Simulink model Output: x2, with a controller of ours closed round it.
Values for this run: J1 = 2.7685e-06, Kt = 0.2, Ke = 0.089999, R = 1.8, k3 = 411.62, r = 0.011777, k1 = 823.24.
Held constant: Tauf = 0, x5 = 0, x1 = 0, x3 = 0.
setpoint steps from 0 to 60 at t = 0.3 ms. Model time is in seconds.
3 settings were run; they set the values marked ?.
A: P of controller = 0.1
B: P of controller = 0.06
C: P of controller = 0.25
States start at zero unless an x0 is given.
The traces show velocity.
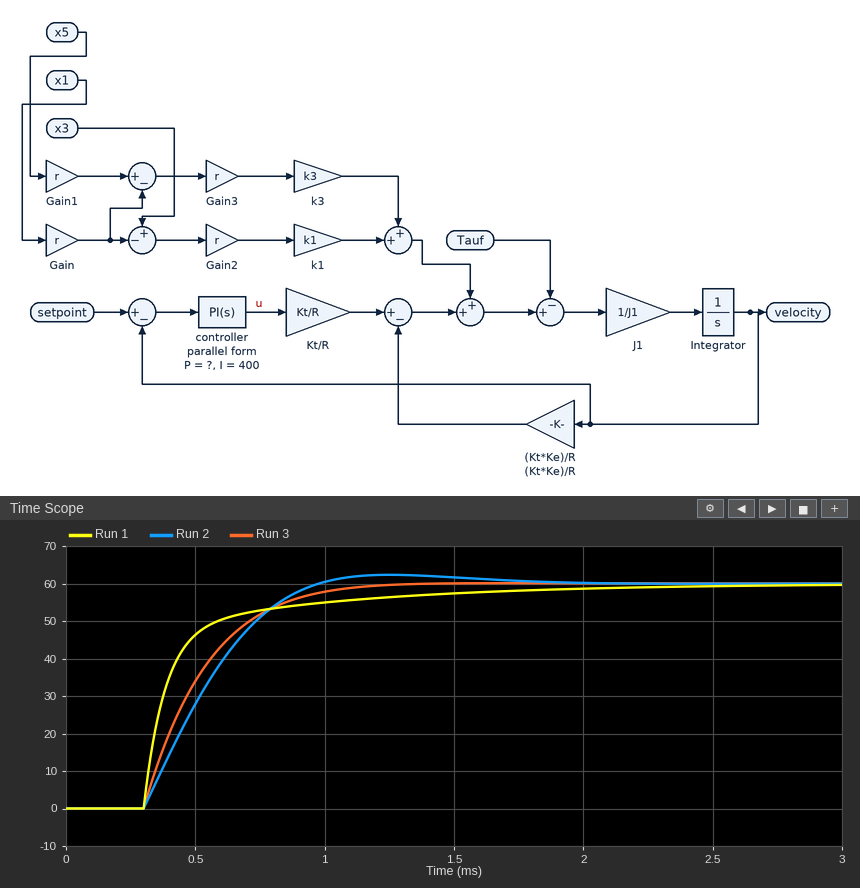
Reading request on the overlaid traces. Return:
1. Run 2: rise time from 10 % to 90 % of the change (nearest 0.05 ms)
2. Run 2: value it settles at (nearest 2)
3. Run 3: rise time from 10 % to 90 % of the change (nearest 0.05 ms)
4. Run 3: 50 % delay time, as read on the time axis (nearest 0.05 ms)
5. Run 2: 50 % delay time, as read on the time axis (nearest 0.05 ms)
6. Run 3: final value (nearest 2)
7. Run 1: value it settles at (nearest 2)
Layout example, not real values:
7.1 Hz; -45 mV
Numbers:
0.45 ms; 60; 0.50 ms; 0.45 ms; 0.50 ms; 60; 60
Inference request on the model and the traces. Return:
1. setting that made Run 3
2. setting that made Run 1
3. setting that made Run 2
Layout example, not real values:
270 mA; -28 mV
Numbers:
A; C; B
